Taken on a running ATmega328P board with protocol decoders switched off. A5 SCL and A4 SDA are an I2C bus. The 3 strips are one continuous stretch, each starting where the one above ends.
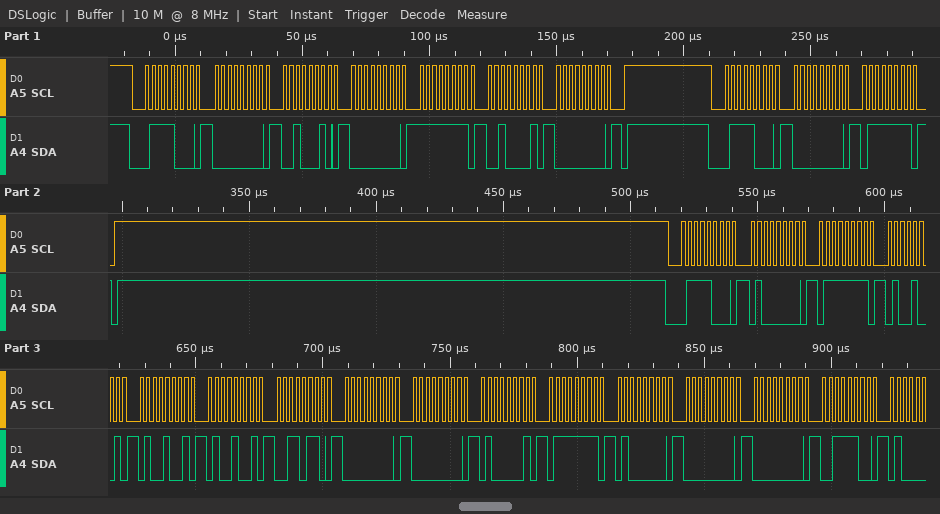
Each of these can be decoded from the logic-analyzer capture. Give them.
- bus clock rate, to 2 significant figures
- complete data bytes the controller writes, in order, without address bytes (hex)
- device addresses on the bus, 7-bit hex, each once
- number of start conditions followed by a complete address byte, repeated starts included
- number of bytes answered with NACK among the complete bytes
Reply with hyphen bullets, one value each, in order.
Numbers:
- 400 kHz
- 00 22 00 FF 21 00 00 7F 40 7F 49 49 49 36 00 00 41 7F 40 00 00 3C
- 0x3C
- 3
- 0
